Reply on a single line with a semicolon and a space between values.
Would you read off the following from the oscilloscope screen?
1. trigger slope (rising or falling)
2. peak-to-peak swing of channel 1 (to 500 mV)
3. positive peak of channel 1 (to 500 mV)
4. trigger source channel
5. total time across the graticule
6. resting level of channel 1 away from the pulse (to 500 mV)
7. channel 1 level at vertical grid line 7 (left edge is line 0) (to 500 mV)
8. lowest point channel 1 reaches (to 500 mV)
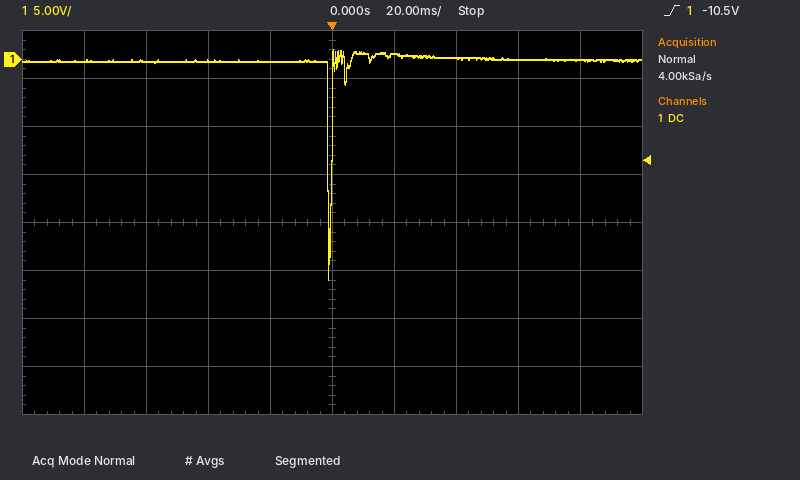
rising; 24.0 V; 1.0 V; channel 1; 200 ms; 0.0 V; 0.0 V; -23.0 V
